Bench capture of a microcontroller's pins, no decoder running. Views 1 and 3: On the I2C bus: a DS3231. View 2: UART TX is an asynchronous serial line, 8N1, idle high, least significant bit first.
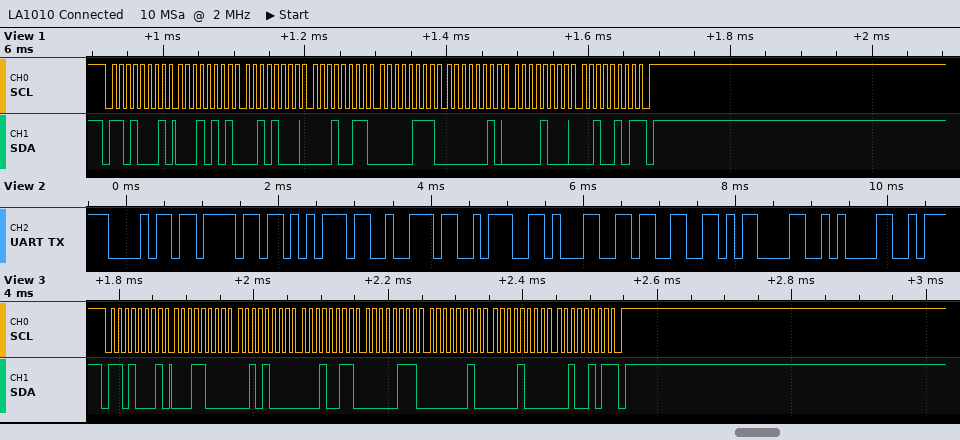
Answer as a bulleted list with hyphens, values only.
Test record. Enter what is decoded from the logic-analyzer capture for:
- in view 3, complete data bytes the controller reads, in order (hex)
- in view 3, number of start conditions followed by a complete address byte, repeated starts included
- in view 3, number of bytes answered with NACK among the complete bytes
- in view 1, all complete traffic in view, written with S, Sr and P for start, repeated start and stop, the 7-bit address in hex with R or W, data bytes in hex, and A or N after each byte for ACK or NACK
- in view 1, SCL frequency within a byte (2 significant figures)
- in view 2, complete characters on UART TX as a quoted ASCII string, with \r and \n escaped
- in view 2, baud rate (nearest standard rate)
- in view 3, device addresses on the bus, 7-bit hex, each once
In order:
- 18 28 13 07 02 08 25
- 1
- 1
- S 68R A 15 A 28 A 13 A 07 A 02 A 08 A 25 N P
- 100 kHz
- "hour:13\r\n"
- 9600 baud
- 0x68
